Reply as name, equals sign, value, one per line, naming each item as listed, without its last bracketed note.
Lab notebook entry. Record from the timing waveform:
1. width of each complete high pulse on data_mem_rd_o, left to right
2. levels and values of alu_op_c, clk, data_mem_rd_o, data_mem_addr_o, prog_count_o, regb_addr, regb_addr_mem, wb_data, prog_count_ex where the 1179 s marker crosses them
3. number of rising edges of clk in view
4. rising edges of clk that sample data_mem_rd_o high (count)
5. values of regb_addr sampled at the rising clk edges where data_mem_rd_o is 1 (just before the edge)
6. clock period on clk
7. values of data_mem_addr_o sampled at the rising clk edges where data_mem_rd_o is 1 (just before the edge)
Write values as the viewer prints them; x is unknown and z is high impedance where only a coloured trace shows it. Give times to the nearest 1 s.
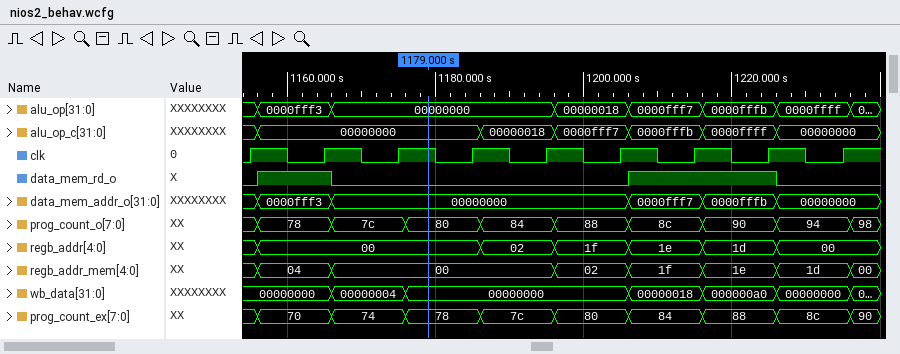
width of each complete high pulse on data_mem_rd_o, left to right = 10 s, 20 s
levels and values of alu_op_c, clk, data_mem_rd_o, data_mem_addr_o, prog_count_o, regb_addr, regb_addr_mem, wb_data, prog_count_ex where the 1179 s marker crosses them = alu_op_c=00000000, clk=1, data_mem_rd_o=0, data_mem_addr_o=00000000, prog_count_o=80, regb_addr=00, regb_addr_mem=00, wb_data=00000000, prog_count_ex=78
number of rising edges of clk in view = 9
rising edges of clk that sample data_mem_rd_o high = 3
values of regb_addr sampled at the rising clk edges where data_mem_rd_o is 1 = 00, 1e, 1d
clock period on clk = 10 s
values of data_mem_addr_o sampled at the rising clk edges where data_mem_rd_o is 1 = 0000fff3, 0000fff7, 0000fffb
